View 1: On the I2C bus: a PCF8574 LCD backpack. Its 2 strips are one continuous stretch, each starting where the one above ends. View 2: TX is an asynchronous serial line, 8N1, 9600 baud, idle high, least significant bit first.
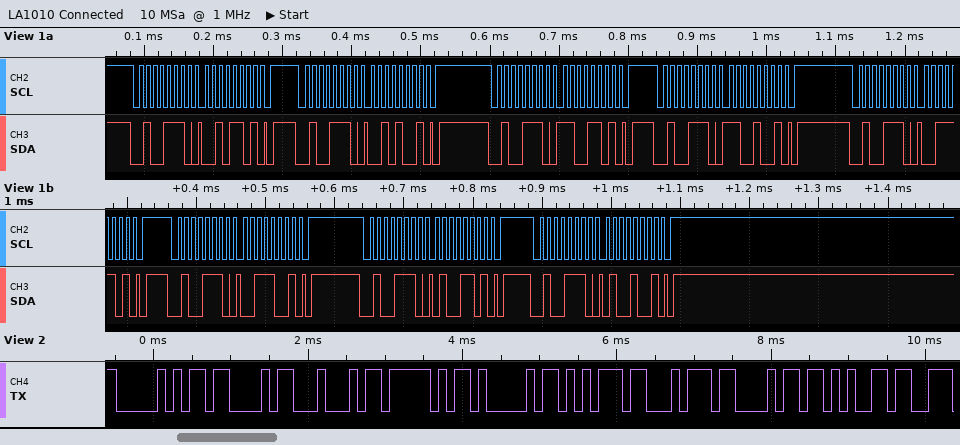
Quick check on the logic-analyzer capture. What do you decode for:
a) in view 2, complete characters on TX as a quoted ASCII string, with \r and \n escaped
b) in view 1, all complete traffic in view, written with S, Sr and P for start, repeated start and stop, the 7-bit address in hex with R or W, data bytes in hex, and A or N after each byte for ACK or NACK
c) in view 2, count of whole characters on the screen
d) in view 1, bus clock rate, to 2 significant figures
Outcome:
"PCD_Authe"
S 27W A 2D A P S 27W A 29 A P S 27W A CD A P S 27W A C9 A P S 27W A 3D A P S 27W A 39 A P S 27W A 4D A P S 27W A 49 A P
9
100 kHz
